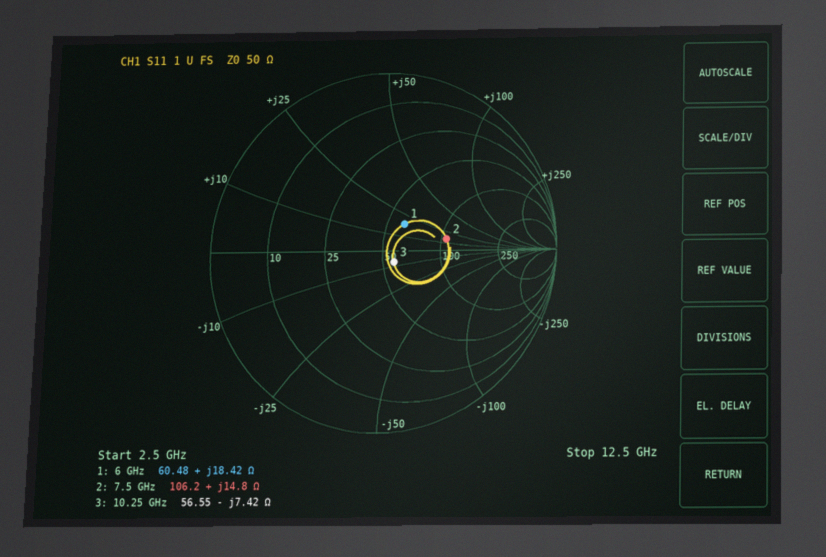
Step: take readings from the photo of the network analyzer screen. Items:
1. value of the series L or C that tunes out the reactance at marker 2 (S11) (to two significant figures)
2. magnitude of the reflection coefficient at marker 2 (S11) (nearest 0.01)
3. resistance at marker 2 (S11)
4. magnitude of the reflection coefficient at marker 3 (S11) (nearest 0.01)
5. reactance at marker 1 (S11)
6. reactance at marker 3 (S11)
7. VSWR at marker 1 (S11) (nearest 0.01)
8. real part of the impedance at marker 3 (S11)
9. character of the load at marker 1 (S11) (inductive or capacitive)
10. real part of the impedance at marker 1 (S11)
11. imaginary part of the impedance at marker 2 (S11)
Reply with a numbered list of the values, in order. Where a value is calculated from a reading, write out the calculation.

1. C = 1/(2π × 7.5 GHz × 14.8 Ω) ≈ 1.4 pF
2. 0.37
3. 106.2 Ω
4. 0.09
5. +18.42 Ω
6. -7.42 Ω
7. 1.47
8. 56.55 Ω
9. inductive
10. 60.48 Ω
11. +14.8 Ω
